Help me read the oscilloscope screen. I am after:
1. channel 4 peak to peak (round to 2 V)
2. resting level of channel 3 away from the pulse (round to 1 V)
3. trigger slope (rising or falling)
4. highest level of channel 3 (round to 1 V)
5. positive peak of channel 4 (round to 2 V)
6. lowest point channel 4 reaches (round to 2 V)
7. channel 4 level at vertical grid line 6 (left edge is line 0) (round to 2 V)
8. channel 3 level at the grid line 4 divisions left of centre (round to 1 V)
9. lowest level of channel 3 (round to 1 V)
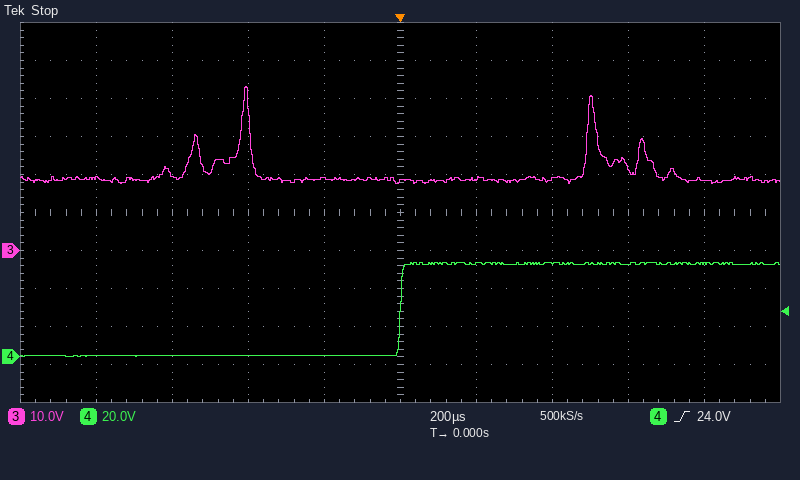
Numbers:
50 V
19 V
rising
43 V
50 V
0 V
50 V
19 V
18 V
